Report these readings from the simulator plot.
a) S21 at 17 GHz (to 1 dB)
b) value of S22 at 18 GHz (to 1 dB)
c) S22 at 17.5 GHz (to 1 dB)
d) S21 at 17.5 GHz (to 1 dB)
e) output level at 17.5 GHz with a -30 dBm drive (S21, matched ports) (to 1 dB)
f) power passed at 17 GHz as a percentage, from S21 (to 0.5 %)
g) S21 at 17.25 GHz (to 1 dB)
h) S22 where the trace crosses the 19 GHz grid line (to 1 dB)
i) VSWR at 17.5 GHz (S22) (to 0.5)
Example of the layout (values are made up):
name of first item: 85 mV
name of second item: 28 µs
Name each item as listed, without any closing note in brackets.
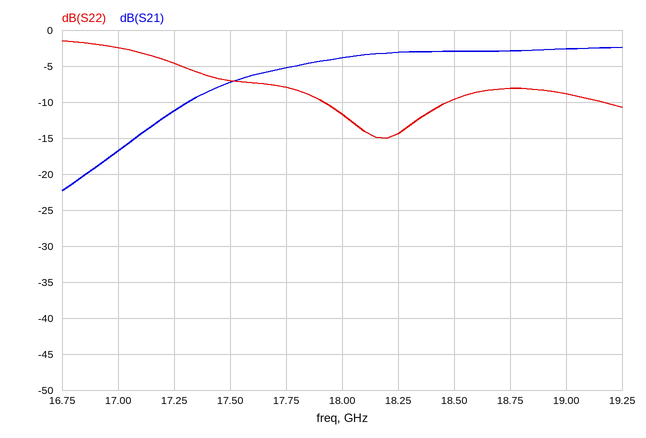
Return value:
S21 at 17 GHz: -17 dB
value of S22 at 18 GHz: -12 dB
S22 at 17.5 GHz: -7 dB
S21 at 17.5 GHz: -7 dB
output level at 17.5 GHz with a -30 dBm drive (S21, matched ports): -37 dBm
power passed at 17 GHz as a percentage, from S21: 2.0 %
S21 at 17.25 GHz: -11 dB
S22 where the trace crosses the 19 GHz grid line: -9 dB
VSWR at 17.5 GHz (S22): 2.5
